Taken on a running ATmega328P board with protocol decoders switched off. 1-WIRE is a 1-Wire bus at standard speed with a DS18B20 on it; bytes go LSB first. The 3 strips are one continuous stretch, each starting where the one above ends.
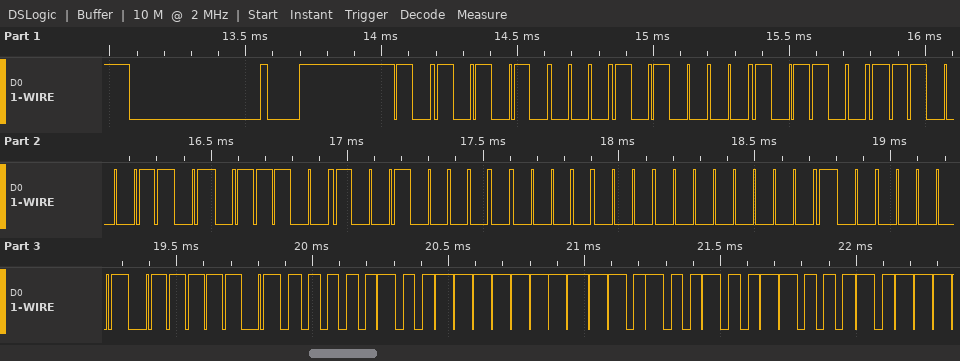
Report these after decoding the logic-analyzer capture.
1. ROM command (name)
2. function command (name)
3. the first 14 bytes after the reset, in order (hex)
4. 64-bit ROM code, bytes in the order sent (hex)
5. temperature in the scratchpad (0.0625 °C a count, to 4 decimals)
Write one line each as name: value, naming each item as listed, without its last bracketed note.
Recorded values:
ROM command: Match ROM
function command: Read Scratchpad
the first 14 bytes after the reset, in order: 55 28 34 C7 3A 09 00 00 81 BE 20 FF 4B 46
64-bit ROM code, bytes in the order sent: 28 34 C7 3A 09 00 00 81
temperature in the scratchpad: -14.0000 °C
